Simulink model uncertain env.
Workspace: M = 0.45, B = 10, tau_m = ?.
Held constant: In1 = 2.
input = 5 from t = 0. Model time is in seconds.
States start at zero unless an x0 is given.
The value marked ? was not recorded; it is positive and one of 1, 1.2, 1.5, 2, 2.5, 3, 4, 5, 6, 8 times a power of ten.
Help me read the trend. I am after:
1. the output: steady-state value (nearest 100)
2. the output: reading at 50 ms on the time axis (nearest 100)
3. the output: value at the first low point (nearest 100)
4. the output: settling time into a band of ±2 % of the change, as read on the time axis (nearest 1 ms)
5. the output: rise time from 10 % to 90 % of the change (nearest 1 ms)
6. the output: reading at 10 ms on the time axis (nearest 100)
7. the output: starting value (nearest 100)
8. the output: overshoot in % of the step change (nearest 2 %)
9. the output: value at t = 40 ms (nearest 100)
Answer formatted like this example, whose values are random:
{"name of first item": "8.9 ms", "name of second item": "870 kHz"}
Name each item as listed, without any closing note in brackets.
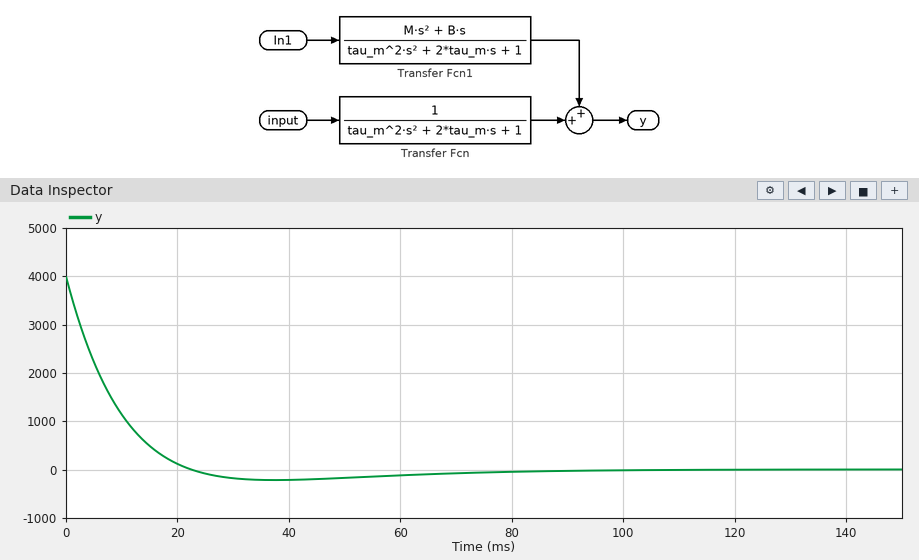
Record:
{"the output: steady-state value": "0", "the output: reading at 50 ms on the time axis": "-200", "the output: value at the first low point": "-200", "the output: settling time into a band of ±2 % of the change, as read on the time axis": "70 ms", "the output: rise time from 10 % to 90 % of the change": "15 ms", "the output: reading at 10 ms on the time axis": "1100", "the output: starting value": "4000", "the output: overshoot in % of the step change": "6 %", "the output: value at t = 40 ms": "-200"}
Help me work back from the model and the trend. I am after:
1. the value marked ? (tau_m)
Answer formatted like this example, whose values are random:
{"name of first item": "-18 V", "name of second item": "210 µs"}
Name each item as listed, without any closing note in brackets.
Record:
{"the value marked ?": "0.015"}
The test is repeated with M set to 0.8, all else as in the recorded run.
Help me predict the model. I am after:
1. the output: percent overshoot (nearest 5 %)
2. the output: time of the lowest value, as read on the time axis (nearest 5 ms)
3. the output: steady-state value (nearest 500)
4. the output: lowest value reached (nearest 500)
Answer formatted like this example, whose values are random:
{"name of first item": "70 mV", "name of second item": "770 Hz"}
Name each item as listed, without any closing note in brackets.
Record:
{"the output: percent overshoot": "10 %", "the output: time of the lowest value, as read on the time axis": "35 ms", "the output: steady-state value": "0", "the output: lowest value reached": "-500"}
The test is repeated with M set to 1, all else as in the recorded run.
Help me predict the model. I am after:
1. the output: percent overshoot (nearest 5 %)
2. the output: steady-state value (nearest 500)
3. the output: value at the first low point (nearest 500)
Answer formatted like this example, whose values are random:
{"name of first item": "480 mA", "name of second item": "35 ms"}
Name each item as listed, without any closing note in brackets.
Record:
{"the output: percent overshoot": "10 %", "the output: steady-state value": "0", "the output: value at the first low point": "-1000"}
